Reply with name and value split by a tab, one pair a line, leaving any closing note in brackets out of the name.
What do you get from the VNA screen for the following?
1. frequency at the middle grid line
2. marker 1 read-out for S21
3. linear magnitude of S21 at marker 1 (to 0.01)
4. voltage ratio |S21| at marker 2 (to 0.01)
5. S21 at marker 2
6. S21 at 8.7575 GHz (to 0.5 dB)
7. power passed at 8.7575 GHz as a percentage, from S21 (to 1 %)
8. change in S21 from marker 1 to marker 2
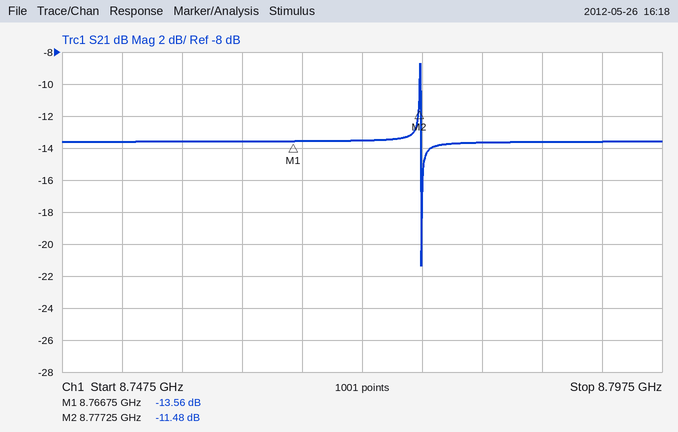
frequency at the middle grid line	8.7725 GHz
marker 1 read-out for S21	-13.56 dB
linear magnitude of S21 at marker 1	0.21
voltage ratio |S21| at marker 2	0.27
S21 at marker 2	-11.48 dB
S21 at 8.7575 GHz	-13.5 dB
power passed at 8.7575 GHz as a percentage, from S21	4 %
change in S21 from marker 1 to marker 2	2.08 dB
